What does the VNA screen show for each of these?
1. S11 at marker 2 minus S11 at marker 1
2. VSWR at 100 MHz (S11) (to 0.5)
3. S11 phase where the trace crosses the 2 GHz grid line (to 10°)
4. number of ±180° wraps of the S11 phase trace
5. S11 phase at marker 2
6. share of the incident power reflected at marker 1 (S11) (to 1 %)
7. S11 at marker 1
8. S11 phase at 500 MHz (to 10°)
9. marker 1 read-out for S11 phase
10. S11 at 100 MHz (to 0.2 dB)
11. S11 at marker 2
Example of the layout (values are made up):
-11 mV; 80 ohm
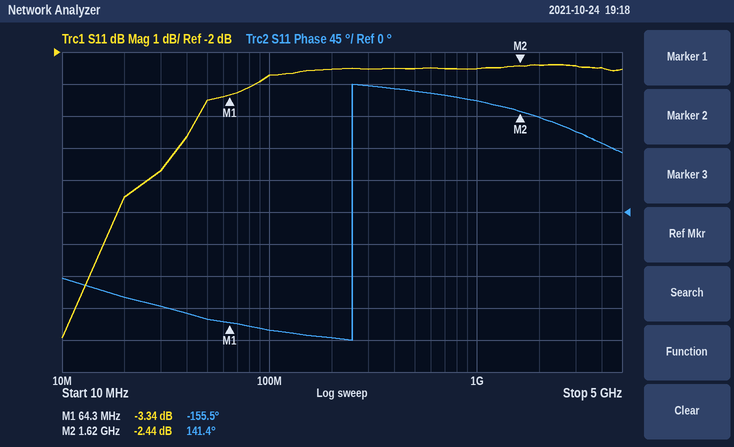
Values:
0.90 dB; 6.5; 130°; 1; 141.4°; 46 %; -3.34 dB; 170°; -155.5°; -2.8 dB; -2.44 dB
